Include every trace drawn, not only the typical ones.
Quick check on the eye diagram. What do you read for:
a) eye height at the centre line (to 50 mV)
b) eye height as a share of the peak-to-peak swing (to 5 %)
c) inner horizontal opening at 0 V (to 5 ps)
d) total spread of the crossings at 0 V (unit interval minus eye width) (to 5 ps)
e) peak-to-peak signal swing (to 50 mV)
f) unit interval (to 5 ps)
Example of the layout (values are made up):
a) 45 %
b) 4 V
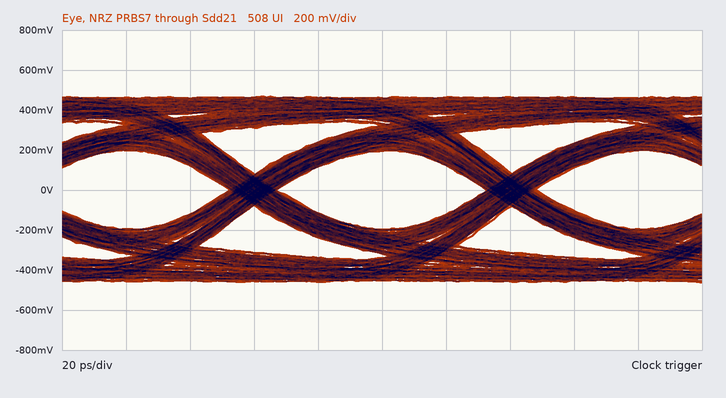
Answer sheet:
a) 400 mV
b) 40 %
c) 65 ps
d) 15 ps
e) 950 mV
f) 80 ps
